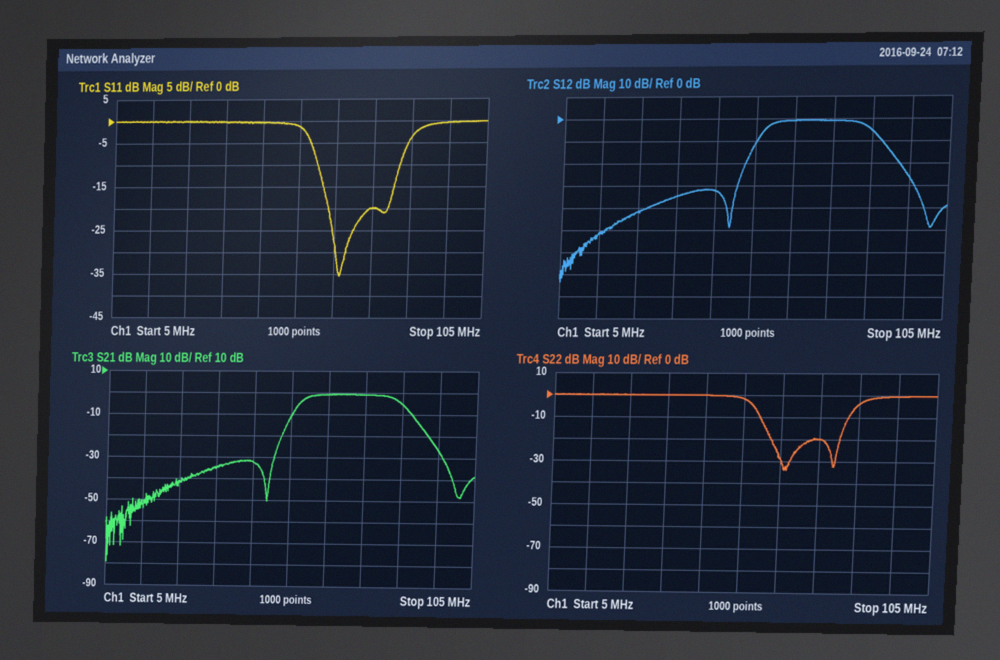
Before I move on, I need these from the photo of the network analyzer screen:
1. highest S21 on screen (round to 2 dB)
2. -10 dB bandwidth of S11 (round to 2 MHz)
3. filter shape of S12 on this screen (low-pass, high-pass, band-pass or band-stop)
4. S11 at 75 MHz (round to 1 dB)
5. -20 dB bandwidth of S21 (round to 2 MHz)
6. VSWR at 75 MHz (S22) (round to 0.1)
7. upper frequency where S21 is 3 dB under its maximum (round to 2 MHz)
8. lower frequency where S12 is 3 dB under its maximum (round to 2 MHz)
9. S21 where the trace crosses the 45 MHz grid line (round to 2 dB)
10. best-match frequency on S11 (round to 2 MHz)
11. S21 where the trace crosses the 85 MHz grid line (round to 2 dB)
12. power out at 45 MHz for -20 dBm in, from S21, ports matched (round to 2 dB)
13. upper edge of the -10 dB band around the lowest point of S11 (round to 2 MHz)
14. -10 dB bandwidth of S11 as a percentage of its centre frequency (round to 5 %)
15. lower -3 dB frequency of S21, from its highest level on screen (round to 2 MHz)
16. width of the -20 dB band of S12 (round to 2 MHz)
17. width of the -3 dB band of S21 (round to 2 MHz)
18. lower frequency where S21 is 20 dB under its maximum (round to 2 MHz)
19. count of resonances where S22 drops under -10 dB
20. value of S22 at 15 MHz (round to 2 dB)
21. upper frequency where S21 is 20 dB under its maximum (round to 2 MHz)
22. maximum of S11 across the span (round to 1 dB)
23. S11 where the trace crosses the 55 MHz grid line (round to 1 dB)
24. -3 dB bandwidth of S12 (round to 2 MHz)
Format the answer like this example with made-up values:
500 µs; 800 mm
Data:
0 dB; 22 MHz; band-pass; -20 dB; 40 MHz; 1.2; 84 MHz; 58 MHz; -32 dB; 66 MHz; -6 dB; -52 dBm; 82 MHz; 30 %; 58 MHz; 40 MHz; 26 MHz; 52 MHz; 2; 0 dB; 92 MHz; 0 dB; -1 dB; 26 MHz
